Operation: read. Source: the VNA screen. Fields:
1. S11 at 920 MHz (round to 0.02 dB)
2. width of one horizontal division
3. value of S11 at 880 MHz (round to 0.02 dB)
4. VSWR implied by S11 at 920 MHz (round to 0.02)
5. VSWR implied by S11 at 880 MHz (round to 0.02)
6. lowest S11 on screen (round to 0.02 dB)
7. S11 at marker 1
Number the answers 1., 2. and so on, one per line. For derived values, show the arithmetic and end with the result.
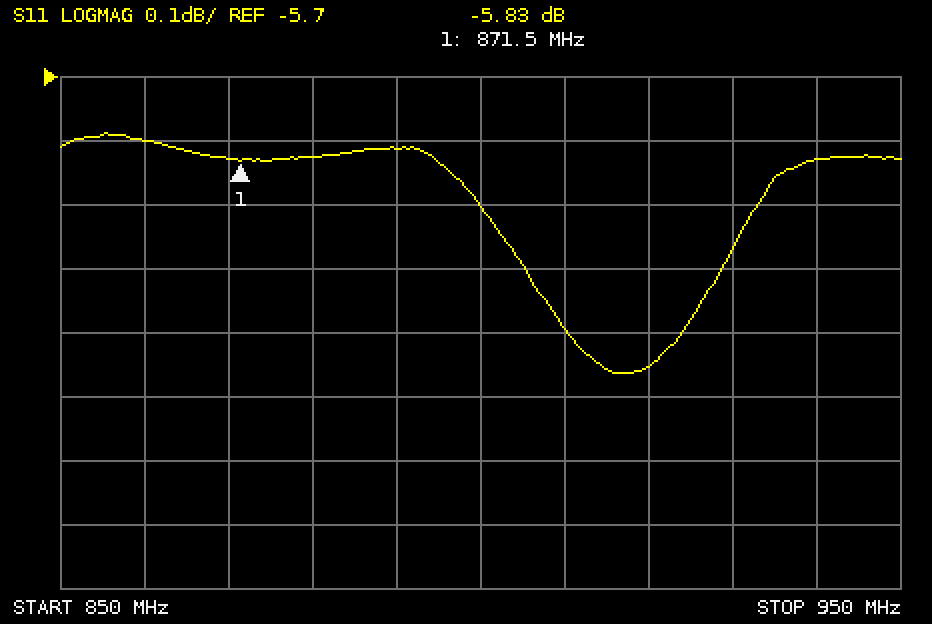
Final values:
1. -6.16 dB
2. 10 MHz
3. -5.82 dB
4. |Γ| = 10^(-6.16/20) = 0.4920; VSWR = (1 + 0.4920)/(1 − 0.4920) ≈ 2.94
5. |Γ| = 10^(-5.82/20) = 0.5117; VSWR = (1 + 0.5117)/(1 − 0.5117) ≈ 3.10
6. -6.16 dB
7. -5.83 dB
